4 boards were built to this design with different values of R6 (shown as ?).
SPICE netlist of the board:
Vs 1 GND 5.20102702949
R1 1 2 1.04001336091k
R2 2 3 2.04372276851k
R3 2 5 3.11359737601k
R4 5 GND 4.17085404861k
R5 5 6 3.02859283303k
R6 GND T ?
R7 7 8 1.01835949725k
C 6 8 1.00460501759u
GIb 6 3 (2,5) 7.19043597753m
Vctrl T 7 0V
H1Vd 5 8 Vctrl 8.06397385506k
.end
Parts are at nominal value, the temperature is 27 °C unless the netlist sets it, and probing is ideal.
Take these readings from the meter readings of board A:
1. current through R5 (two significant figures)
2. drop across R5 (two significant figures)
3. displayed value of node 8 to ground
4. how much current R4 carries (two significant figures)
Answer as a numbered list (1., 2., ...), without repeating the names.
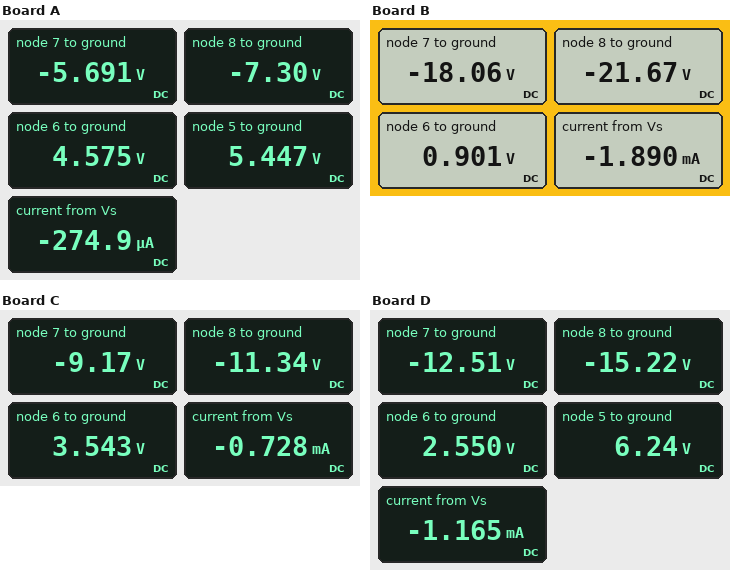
1. 290 µA
2. 870 mV
3. -7.30 V
4. 1.3 mA
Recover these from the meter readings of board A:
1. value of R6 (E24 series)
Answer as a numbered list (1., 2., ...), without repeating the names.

1. 3.6 kΩ
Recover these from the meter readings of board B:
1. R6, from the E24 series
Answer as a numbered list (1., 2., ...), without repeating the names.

1. 5.1 kΩ
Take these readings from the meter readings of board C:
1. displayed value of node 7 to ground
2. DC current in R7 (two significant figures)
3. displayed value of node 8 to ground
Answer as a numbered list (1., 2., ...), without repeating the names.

1. -9.17 V
2. 2.1 mA
3. -11.34 V
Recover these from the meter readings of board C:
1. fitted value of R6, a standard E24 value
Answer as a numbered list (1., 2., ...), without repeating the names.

1. 4.3 kΩ
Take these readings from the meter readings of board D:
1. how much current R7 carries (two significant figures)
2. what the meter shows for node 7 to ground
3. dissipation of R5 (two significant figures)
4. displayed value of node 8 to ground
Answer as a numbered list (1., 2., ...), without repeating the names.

1. 2.7 mA
2. -12.51 V
3. 4.5 mW
4. -15.22 V
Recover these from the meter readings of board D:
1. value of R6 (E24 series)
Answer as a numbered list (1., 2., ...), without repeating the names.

1. 4.7 kΩ
